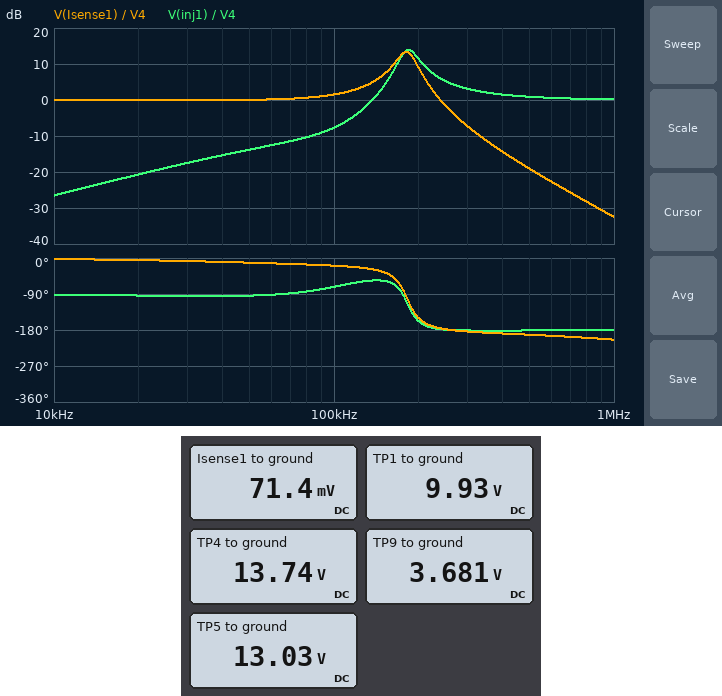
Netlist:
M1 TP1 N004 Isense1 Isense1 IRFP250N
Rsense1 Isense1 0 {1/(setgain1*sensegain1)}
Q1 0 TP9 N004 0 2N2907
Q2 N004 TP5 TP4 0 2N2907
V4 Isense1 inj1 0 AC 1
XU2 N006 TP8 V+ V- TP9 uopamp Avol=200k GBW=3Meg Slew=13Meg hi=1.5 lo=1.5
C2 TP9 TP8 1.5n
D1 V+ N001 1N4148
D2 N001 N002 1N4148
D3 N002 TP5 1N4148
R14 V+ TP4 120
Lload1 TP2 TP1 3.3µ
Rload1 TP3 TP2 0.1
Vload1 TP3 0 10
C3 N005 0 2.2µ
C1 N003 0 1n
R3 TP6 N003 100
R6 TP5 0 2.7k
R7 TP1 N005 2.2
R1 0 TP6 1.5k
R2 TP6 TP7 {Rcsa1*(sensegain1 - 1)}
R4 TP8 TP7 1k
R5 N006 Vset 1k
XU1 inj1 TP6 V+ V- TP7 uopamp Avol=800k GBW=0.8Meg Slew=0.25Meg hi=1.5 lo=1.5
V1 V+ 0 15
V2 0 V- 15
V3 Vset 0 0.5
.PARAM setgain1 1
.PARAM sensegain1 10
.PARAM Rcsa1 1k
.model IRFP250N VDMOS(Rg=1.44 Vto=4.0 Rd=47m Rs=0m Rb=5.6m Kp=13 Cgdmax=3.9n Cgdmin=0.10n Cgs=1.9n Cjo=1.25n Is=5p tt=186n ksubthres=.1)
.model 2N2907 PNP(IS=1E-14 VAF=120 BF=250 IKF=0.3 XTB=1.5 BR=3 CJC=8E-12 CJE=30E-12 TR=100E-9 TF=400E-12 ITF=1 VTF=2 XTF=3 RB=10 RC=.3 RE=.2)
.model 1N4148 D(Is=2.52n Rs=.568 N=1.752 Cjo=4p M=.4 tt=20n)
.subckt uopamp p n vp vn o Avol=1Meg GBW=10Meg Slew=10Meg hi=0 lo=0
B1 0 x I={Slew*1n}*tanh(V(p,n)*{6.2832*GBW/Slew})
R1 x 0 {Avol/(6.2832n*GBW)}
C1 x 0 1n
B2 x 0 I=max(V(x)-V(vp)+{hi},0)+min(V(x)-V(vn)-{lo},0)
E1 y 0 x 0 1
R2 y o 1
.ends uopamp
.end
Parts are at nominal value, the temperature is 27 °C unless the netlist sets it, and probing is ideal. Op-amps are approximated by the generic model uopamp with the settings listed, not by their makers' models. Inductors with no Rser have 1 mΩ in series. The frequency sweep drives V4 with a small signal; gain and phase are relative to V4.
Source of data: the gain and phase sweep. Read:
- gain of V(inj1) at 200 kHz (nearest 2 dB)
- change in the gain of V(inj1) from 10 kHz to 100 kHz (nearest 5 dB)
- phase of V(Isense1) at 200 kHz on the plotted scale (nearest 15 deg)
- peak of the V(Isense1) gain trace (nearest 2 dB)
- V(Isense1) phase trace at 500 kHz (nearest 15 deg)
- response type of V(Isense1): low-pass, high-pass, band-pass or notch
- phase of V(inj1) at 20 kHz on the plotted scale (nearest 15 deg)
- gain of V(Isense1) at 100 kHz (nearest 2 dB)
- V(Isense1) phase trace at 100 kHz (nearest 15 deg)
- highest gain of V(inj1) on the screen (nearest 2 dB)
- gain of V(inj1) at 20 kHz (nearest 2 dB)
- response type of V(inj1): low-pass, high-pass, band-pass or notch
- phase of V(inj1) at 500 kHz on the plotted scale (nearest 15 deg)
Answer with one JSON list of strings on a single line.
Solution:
["12 dB", "20 dB", "-150 deg", "14 dB", "-195 deg", "low-pass", "-90 deg", "2 dB", "-15 deg", "14 dB", "-20 dB", "high-pass", "-180 deg"]
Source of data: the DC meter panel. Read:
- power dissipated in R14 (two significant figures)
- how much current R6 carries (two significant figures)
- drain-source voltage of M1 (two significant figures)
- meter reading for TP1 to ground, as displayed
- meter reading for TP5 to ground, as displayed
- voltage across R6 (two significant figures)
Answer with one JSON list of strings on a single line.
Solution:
["13 mW", "4.8 mA", "9.9 V", "9.93 V", "13.03 V", "13 V"]
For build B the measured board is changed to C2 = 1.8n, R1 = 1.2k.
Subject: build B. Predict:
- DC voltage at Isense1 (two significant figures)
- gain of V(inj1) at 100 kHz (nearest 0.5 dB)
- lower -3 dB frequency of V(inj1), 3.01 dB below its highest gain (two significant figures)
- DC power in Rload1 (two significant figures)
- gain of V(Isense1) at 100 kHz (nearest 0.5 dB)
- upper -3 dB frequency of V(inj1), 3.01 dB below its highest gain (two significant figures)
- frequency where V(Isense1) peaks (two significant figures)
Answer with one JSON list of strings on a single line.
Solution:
["59 mV", "-4.0 dB", "150 kHz", "35 mW", "2.5 dB", "190 kHz", "160 kHz"]
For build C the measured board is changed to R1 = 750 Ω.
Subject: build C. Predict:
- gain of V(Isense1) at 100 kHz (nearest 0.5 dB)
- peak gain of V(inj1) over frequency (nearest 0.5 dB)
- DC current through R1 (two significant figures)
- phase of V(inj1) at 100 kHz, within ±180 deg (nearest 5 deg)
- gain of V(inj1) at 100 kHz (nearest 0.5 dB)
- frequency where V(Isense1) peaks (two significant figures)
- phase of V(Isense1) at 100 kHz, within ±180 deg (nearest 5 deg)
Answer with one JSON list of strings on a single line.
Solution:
["4.0 dB", "11.5 dB", "51 µA", "-55 deg", "-1.5 dB", "150 kHz", "-25 deg"]
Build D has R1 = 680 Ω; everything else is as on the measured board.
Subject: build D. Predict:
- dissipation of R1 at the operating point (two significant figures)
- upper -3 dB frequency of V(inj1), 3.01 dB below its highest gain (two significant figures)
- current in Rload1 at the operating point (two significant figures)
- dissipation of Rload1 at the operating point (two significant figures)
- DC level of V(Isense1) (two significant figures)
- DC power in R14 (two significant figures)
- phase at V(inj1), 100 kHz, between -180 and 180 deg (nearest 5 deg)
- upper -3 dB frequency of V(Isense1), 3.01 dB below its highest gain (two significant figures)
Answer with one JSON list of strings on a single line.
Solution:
["1.8 µW", "170 kHz", "350 mA", "12 mW", "35 mV", "13 mW", "-55 deg", "160 kHz"]
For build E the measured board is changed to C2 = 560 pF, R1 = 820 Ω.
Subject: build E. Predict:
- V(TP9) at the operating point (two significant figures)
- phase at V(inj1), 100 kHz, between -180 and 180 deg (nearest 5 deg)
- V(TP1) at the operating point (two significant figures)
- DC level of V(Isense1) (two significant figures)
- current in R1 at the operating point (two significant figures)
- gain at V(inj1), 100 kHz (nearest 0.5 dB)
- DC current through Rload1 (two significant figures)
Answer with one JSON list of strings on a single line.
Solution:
["3.6 V", "-40 deg", "10 V", "42 mV", "51 µA", "-13.0 dB", "420 mA"]
